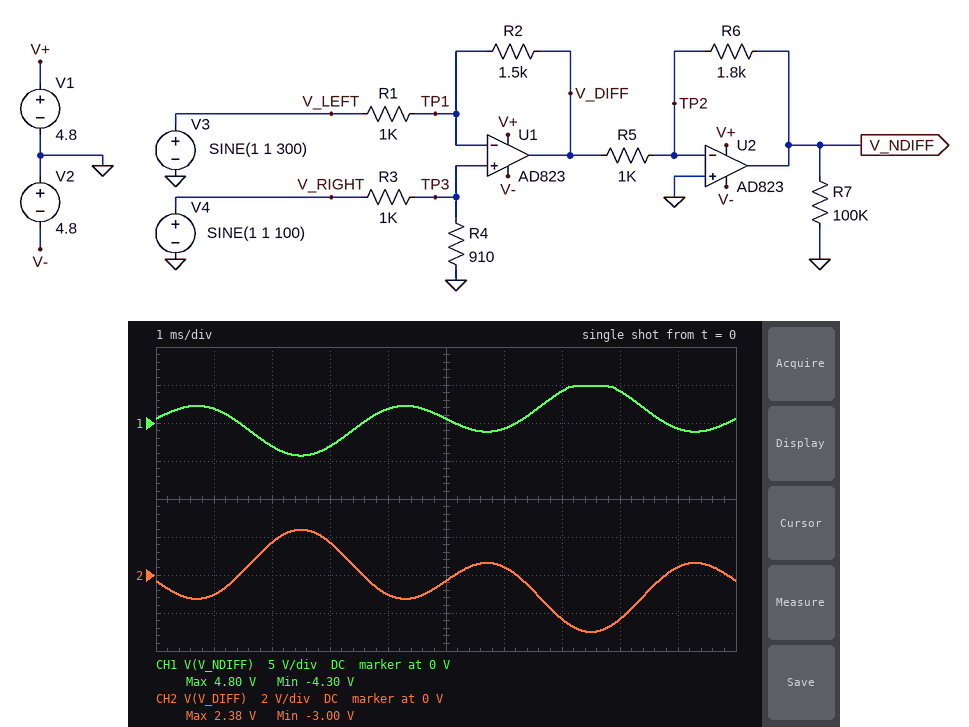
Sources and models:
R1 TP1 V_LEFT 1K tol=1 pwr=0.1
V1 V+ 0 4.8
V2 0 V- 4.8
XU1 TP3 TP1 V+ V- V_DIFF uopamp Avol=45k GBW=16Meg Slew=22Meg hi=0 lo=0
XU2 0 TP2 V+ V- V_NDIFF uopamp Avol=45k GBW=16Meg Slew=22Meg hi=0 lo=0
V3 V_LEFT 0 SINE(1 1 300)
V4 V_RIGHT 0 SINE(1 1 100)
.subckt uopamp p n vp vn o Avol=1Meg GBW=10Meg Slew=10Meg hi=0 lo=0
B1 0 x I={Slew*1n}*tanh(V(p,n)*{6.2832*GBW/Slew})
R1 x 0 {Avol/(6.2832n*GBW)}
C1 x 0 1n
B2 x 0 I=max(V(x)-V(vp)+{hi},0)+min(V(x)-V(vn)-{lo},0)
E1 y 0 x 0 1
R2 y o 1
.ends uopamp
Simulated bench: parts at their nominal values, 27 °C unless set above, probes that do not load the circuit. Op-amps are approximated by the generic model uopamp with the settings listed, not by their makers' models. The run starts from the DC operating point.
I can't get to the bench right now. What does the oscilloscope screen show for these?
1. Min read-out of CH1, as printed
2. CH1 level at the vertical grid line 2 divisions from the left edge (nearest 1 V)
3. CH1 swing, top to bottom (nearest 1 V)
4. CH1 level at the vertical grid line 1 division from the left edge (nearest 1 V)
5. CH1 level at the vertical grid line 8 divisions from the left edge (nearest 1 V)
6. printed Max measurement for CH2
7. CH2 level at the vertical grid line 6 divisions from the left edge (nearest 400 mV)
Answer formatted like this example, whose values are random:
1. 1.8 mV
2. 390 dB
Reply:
1. -4.30 V
2. -3 V
3. 9 V
4. 2 V
5. 4 V
6. 2.38 V
7. 400 mV
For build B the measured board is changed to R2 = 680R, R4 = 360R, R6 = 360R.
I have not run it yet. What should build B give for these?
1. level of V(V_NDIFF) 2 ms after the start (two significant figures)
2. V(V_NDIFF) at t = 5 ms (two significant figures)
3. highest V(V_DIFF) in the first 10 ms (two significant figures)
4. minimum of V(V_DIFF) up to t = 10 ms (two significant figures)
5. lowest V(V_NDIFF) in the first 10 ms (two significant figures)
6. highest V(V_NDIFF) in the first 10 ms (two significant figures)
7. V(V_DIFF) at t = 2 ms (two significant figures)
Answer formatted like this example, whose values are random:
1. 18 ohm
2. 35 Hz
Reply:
1. -210 mV
2. 85 mV
3. 890 mV
4. -1.4 V
5. -320 mV
6. 490 mV
7. 590 mV
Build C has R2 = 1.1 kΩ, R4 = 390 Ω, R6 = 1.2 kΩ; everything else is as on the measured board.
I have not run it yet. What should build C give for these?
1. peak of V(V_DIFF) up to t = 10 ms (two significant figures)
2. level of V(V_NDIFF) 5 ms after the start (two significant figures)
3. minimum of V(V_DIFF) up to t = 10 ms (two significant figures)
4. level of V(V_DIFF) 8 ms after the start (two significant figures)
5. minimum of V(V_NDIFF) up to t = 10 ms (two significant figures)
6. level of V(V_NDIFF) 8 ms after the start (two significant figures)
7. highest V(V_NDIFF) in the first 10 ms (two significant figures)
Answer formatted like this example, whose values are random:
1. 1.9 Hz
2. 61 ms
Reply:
1. 1.2 V
2. 610 mV
3. -2.2 V
4. -1.7 V
5. -1.4 V
6. 2.1 V
7. 2.6 V
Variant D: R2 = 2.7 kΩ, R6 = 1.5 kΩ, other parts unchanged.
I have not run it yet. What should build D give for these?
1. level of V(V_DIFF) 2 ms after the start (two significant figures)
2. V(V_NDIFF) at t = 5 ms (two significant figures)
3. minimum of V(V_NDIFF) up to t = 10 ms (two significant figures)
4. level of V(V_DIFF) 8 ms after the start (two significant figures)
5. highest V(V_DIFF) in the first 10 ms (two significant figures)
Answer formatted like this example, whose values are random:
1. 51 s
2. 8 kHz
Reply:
1. 2.3 V
2. 1.4 V
3. -4.8 V
4. -4.2 V
5. 3.5 V
